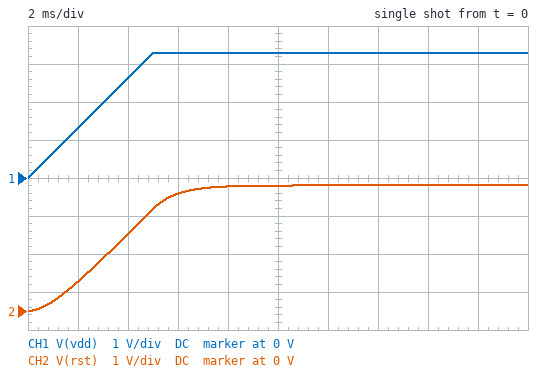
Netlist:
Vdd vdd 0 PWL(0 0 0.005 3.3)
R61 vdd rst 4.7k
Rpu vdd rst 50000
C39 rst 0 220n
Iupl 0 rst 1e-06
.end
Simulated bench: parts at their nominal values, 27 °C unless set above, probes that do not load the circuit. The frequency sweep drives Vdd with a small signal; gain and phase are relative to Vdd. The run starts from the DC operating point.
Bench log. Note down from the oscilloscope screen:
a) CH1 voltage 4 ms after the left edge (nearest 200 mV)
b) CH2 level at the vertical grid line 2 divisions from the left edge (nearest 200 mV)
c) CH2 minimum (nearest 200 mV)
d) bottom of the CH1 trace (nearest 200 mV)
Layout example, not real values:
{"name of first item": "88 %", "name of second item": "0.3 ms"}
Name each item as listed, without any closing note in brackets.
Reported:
{"CH1 voltage 4 ms after the left edge": "2.6 V", "CH2 level at the vertical grid line 2 divisions from the left edge": "2.0 V", "CH2 minimum": "0 V", "bottom of the CH1 trace": "0 V"}
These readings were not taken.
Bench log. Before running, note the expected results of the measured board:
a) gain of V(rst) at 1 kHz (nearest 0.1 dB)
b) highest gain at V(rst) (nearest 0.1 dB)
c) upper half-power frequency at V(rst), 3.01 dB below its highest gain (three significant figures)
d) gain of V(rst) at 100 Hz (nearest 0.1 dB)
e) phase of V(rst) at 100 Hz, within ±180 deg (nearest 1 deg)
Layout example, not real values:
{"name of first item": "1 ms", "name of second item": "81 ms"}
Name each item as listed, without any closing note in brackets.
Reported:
{"gain of V(rst) at 1 kHz": "-15.6 dB", "highest gain at V(rst)": "0 dB", "upper half-power frequency at V(rst), 3.01 dB below its highest gain": "168 Hz", "gain of V(rst) at 100 Hz": "-1.3 dB", "phase of V(rst) at 100 Hz, within ±180 deg": "-31 deg"}
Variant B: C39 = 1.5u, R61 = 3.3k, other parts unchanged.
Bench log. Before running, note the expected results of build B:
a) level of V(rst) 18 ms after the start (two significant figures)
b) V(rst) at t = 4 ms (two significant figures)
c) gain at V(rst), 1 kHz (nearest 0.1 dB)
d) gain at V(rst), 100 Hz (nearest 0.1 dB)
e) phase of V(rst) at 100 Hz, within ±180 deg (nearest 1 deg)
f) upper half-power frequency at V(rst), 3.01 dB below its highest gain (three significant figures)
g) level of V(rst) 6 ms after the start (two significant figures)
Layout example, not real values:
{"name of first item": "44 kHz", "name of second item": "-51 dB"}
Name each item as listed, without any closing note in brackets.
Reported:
{"level of V(rst) 18 ms after the start": "3.2 V", "V(rst) at t = 4 ms": "870 mV", "gain at V(rst), 1 kHz": "-29.3 dB", "gain at V(rst), 100 Hz": "-9.8 dB", "phase of V(rst) at 100 Hz, within ±180 deg": "-71 deg", "upper half-power frequency at V(rst), 3.01 dB below its highest gain": "34.3 Hz", "level of V(rst) 6 ms after the start": "1.7 V"}
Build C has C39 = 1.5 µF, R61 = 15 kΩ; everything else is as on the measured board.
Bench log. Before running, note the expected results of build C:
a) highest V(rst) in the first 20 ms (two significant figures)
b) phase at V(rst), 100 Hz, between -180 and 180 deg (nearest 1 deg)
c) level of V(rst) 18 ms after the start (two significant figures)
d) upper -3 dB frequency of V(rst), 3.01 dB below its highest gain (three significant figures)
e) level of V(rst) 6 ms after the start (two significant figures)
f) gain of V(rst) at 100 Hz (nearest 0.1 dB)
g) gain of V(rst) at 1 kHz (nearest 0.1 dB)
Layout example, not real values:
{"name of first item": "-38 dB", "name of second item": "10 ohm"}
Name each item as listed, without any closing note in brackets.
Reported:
{"highest V(rst) in the first 20 ms": "2.1 V", "phase at V(rst), 100 Hz, between -180 and 180 deg": "-85 deg", "level of V(rst) 18 ms after the start": "2.0 V", "upper -3 dB frequency of V(rst), 3.01 dB below its highest gain": "9.20 Hz", "level of V(rst) 6 ms after the start": "610 mV", "gain of V(rst) at 100 Hz": "-20.8 dB", "gain of V(rst) at 1 kHz": "-40.7 dB"}
